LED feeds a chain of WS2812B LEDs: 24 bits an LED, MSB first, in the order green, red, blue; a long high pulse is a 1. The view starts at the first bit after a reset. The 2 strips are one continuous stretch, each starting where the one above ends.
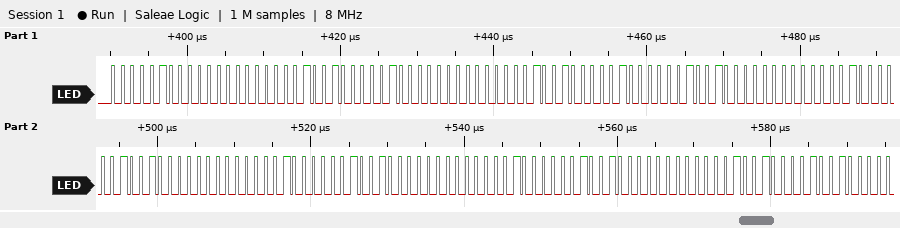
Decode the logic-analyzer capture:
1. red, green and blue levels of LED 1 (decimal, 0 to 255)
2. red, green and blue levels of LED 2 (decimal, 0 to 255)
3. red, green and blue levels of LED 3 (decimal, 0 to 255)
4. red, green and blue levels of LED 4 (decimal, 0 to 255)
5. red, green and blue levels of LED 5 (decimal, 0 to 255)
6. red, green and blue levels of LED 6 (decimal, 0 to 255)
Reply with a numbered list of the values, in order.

1. 0, 4, 9
2. 0, 4, 9
3. 9, 4, 0
4. 9, 4, 0
5. 9, 4, 0
6. 9, 4, 0
